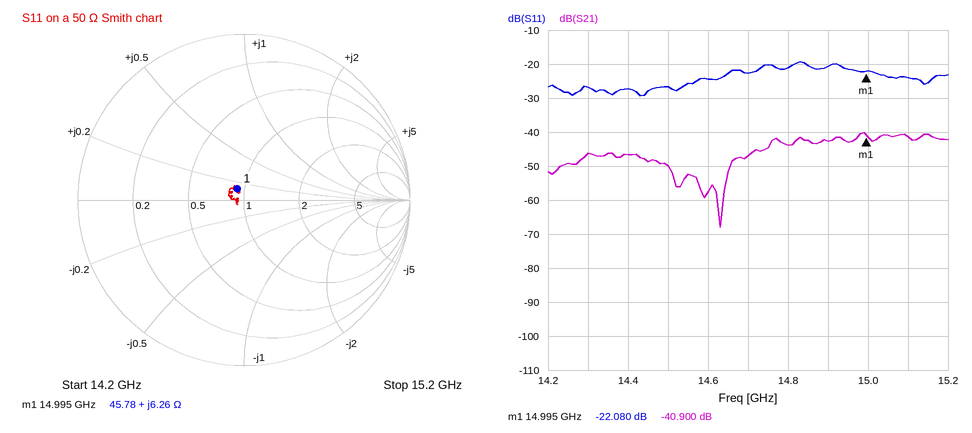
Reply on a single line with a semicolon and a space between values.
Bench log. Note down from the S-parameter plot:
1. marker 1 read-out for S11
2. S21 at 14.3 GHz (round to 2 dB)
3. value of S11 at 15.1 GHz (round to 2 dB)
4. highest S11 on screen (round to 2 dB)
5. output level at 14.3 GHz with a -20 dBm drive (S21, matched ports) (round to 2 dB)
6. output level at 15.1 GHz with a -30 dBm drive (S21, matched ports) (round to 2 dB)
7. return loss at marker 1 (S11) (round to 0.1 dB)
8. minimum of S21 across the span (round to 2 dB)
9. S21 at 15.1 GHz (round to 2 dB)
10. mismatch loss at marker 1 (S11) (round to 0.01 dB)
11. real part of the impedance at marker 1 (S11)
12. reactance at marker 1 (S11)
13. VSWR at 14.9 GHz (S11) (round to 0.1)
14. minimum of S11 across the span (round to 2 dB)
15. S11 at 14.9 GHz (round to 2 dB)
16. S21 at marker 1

-22.080 dB; -46 dB; -24 dB; -20 dB; -66 dBm; -72 dBm; 22.1 dB; -68 dB; -42 dB; 0.03 dB; 45.78 Ω; +6.26 Ω; 1.2; -30 dB; -20 dB; -40.900 dB
